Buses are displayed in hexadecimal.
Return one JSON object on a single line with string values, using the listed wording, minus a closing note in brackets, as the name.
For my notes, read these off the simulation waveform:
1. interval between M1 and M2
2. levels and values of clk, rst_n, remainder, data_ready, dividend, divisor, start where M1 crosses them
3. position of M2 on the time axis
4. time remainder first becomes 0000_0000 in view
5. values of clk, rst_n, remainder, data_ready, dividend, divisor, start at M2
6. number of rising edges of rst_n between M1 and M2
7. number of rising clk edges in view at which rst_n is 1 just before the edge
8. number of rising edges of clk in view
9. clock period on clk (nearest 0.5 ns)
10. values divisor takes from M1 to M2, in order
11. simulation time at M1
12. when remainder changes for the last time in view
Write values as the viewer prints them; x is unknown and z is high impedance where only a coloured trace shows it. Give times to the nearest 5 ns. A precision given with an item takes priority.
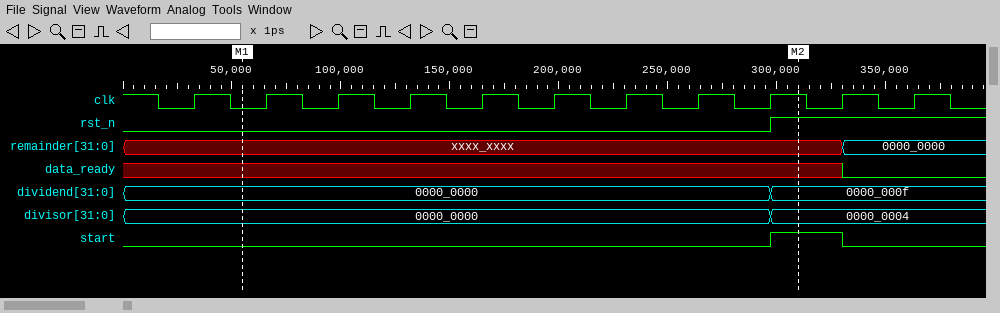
{"interval between M1 and M2": "255 ns", "levels and values of clk, rst_n, remainder, data_ready, dividend, divisor, start where M1 crosses them": "clk=0, rst_n=0, remainder=xxxx_xxxx, data_ready=x, dividend=0000_0000, divisor=0000_0000, start=0", "position of M2 on the time axis": "310 ns", "time remainder first becomes 0000_0000 in view": "330 ns", "values of clk, rst_n, remainder, data_ready, dividend, divisor, start at M2": "clk=1, rst_n=1, remainder=xxxx_xxxx, data_ready=x, dividend=0000_000f, divisor=0000_0004, start=1", "number of rising edges of rst_n between M1 and M2": "1", "number of rising clk edges in view at which rst_n is 1 just before the edge": "2", "number of rising edges of clk in view": "11", "clock period on clk": "33 ns", "values divisor takes from M1 to M2, in order": "0000_0000, 0000_0004", "simulation time at M1": "55 ns", "when remainder changes for the last time in view": "330 ns"}
